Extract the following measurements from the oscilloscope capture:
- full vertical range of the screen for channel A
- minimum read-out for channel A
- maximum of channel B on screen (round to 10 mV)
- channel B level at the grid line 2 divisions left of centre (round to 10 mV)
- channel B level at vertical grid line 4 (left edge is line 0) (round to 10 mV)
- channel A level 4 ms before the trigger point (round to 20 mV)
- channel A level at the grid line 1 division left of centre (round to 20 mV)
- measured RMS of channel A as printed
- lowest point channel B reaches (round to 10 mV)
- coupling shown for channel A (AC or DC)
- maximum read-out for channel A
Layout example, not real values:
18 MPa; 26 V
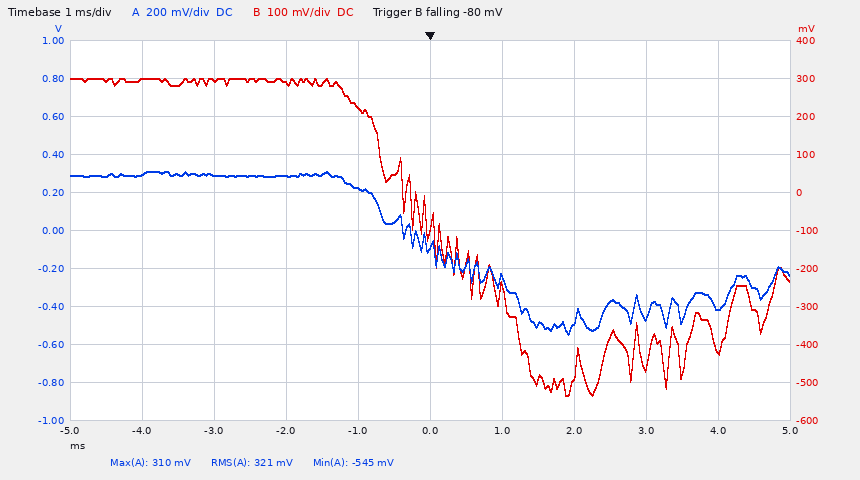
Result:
2 V; -545 mV; 300 mV; 290 mV; 220 mV; 300 mV; 220 mV; 321 mV; -530 mV; DC; 310 mV
